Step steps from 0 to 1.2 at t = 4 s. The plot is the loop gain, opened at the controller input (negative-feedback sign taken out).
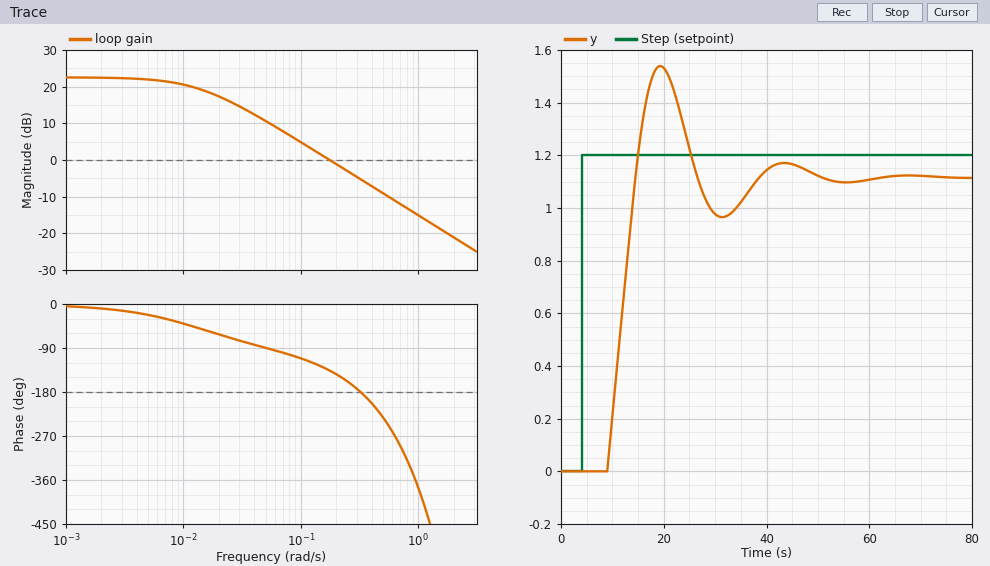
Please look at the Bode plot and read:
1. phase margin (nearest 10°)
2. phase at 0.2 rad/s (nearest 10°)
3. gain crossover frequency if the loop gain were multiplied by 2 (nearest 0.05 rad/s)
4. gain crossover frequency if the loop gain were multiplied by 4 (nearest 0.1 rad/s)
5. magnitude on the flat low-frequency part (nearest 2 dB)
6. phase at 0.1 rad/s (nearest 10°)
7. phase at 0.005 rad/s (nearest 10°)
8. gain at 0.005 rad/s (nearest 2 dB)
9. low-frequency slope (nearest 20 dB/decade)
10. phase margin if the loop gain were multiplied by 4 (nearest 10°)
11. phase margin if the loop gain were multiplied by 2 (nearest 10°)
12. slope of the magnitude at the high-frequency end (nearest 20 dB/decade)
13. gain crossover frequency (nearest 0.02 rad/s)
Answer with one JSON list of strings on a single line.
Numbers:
["40°", "-140°", "0.35 rad/s", "0.7 rad/s", "22 dB", "-110°", "-20°", "22 dB", "0 dB/decade", "-110°", "-10°", "-20 dB/decade", "0.18 rad/s"]
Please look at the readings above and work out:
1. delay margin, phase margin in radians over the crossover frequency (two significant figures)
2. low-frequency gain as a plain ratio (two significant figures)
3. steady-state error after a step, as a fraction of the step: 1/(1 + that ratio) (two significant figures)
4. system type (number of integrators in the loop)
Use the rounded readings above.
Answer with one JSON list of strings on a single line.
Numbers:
["3.9 s", "13", "0.071", "0"]
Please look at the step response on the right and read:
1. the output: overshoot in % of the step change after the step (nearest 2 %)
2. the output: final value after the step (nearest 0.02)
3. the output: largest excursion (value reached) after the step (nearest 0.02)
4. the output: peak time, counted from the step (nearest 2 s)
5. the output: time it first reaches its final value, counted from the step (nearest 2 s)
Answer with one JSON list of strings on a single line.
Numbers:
["38 %", "1.12", "1.54", "16 s", "10 s"]
